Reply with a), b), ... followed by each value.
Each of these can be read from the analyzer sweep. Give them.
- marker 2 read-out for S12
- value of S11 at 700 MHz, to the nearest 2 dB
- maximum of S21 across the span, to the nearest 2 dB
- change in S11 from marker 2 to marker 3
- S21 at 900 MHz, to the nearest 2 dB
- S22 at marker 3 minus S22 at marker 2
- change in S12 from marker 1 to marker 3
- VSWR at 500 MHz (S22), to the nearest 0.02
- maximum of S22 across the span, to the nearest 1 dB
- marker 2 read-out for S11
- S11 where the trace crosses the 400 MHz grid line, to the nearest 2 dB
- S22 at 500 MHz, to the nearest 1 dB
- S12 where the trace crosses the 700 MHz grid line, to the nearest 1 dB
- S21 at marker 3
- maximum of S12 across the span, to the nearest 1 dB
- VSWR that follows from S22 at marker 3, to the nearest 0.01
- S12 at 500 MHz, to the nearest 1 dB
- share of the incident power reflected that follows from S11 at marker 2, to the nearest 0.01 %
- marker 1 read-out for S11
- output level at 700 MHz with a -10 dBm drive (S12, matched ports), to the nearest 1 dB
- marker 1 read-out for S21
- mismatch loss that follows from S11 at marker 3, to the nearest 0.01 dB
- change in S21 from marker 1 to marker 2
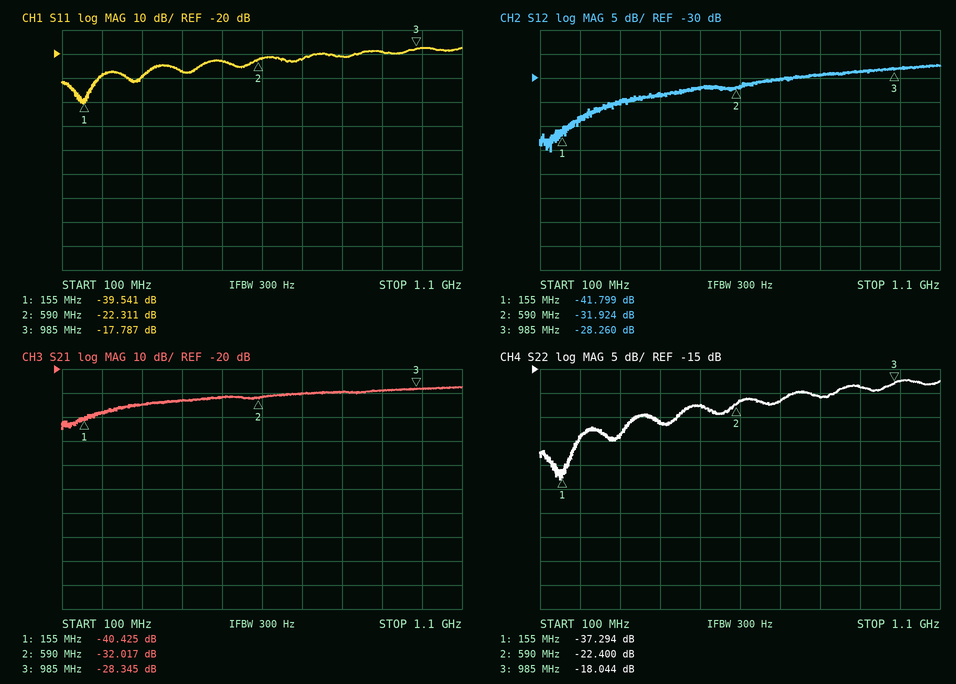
a) -31.924 dB
b) -22 dB
c) -28 dB
d) 4.524 dB
e) -28 dB
f) 4.356 dB
g) 13.539 dB
h) 1.16
i) -17 dB
j) -22.311 dB
k) -28 dB
l) -23 dB
m) -30 dB
n) -28.345 dB
o) -27 dB
p) 1.29
q) -32 dB
r) 0.59 %
s) -39.541 dB
t) -40 dBm
u) -40.425 dB
v) 0.07 dB
w) 8.408 dB
